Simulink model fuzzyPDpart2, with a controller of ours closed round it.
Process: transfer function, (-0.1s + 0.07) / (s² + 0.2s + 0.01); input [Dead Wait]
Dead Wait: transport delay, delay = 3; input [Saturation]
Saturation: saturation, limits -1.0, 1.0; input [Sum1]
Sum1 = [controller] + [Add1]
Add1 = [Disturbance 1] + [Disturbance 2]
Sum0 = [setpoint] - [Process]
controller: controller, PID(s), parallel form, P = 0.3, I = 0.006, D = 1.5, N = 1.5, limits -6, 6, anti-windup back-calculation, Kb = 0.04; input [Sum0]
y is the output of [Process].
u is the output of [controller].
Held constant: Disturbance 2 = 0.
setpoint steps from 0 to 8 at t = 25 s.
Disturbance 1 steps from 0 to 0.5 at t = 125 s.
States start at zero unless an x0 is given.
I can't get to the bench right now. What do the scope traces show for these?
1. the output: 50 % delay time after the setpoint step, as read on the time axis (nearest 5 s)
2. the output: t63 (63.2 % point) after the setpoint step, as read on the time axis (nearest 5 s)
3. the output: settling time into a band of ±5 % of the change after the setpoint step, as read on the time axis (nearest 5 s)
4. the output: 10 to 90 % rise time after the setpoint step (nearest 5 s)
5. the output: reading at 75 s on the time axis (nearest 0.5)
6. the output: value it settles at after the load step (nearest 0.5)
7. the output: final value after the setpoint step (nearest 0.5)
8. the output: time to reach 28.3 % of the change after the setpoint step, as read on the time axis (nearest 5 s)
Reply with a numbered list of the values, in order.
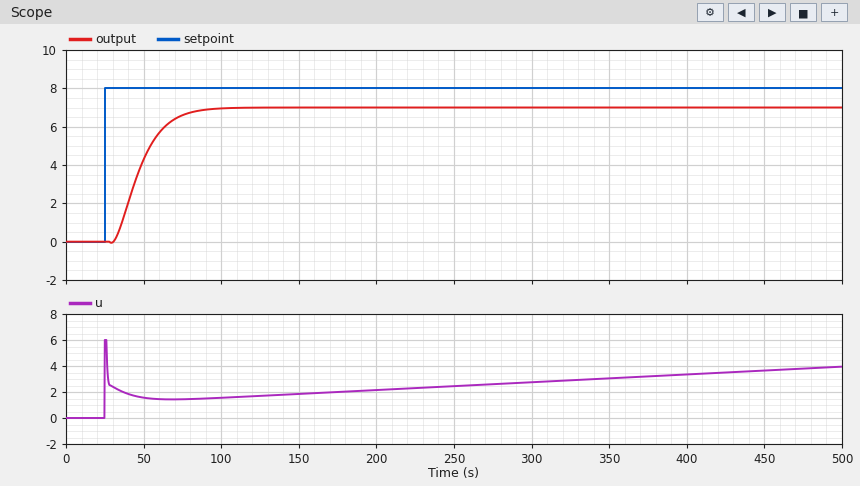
1. 45 s
2. 50 s
3. 75 s
4. 35 s
5. 6.5
6. 7.0
7. 7.0
8. 40 s
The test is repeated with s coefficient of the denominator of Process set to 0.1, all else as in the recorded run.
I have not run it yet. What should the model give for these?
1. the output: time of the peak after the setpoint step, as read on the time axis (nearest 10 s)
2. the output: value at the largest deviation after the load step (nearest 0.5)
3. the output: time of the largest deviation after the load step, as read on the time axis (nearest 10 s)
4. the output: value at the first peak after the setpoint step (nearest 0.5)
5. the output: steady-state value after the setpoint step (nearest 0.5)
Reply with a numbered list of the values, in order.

1. 60 s
2. 7.0
3. 150 s
4. 7.5
5. 7.0
